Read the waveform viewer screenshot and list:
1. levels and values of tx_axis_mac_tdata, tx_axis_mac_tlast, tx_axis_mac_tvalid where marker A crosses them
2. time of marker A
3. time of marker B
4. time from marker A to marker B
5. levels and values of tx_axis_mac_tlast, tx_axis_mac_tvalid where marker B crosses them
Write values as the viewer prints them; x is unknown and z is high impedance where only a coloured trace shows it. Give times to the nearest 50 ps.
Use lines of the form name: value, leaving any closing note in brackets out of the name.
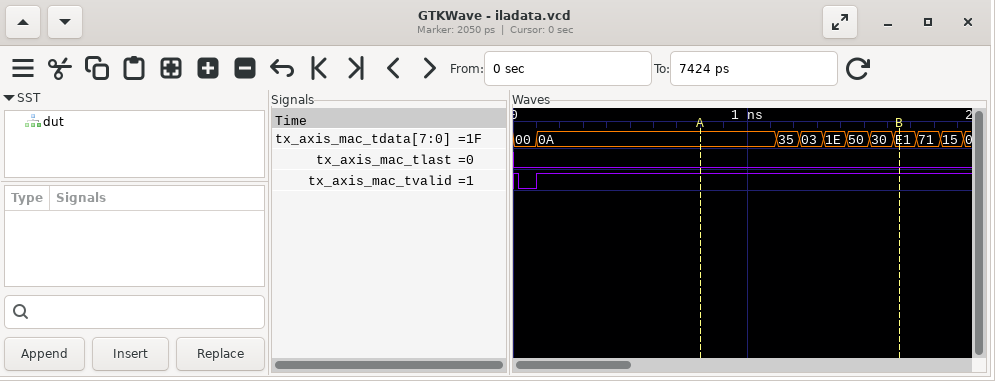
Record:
levels and values of tx_axis_mac_tdata, tx_axis_mac_tlast, tx_axis_mac_tvalid where marker A crosses them: tx_axis_mac_tdata=0A, tx_axis_mac_tlast=0, tx_axis_mac_tvalid=1
time of marker A: 800 ps
time of marker B: 1650 ps
time from marker A to marker B: 850 ps
levels and values of tx_axis_mac_tlast, tx_axis_mac_tvalid where marker B crosses them: tx_axis_mac_tlast=0, tx_axis_mac_tvalid=1
